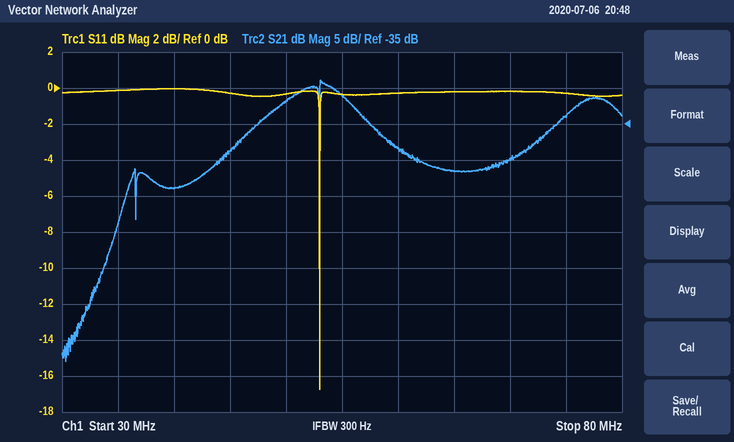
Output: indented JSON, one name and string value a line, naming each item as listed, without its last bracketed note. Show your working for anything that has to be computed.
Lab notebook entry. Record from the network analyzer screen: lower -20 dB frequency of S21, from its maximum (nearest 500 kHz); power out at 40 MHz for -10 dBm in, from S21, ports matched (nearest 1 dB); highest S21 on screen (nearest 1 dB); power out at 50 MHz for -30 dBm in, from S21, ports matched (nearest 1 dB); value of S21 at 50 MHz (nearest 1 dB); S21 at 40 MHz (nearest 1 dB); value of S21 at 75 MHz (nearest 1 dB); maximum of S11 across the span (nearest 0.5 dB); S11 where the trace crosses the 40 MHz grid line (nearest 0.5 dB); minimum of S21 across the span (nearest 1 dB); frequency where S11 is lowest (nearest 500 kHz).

{
  "lower -20 dB frequency of S21, from its maximum": "35.0 MHz",
  "power out at 40 MHz for -10 dBm in, from S21, ports matched": "-10 dBm + (-44 dB) = -54 dBm",
  "highest S21 on screen": "-29 dB",
  "power out at 50 MHz for -30 dBm in, from S21, ports matched": "-30 dBm + (-32 dB) = -62 dBm",
  "value of S21 at 50 MHz": "-32 dB",
  "S21 at 40 MHz": "-44 dB",
  "value of S21 at 75 MHz": "-34 dB",
  "maximum of S11 across the span": "0.0 dB",
  "S11 where the trace crosses the 40 MHz grid line": "0.0 dB",
  "minimum of S21 across the span": "-68 dB",
  "frequency where S11 is lowest": "53.0 MHz"
}
